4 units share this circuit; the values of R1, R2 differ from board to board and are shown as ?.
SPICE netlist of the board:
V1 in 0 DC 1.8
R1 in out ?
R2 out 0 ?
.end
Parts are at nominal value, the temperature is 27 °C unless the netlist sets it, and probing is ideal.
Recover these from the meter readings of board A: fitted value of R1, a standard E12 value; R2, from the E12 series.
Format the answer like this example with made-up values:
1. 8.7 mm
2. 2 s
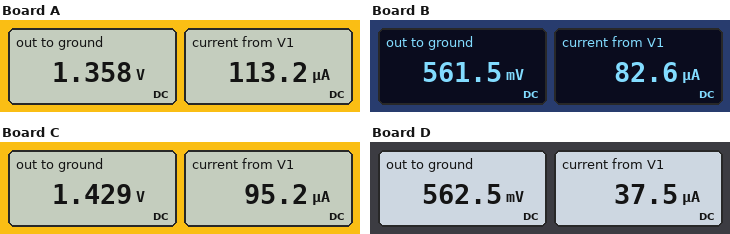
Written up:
1. 3.9 kΩ
2. 12 kΩ
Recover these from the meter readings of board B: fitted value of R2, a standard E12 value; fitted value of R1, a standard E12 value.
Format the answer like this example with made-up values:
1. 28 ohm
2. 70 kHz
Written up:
1. 6.8 kΩ
2. 15 kΩ
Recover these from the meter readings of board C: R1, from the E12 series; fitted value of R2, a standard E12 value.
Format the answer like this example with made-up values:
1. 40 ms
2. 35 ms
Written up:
1. 3.9 kΩ
2. 15 kΩ
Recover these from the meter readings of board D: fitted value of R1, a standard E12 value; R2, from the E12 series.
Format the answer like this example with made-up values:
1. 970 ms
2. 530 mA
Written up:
1. 33 kΩ
2. 15 kΩ
